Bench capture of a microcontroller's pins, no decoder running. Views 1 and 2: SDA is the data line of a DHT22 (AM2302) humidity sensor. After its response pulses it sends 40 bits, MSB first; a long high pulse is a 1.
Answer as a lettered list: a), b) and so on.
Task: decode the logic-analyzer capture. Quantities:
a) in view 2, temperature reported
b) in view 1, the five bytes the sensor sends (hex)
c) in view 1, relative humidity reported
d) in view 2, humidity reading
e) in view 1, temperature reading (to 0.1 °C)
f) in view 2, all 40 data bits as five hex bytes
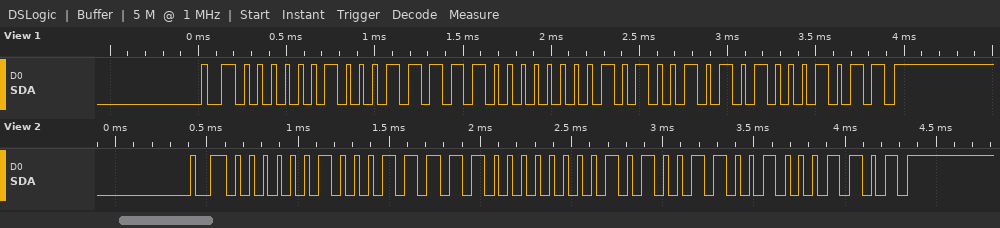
a) 33.2 °C
b) 02 3E 01 4A 8B
c) 57.4 %
d) 57.4 %
e) 33.0 °C
f) 02 3E 01 4C 8D
